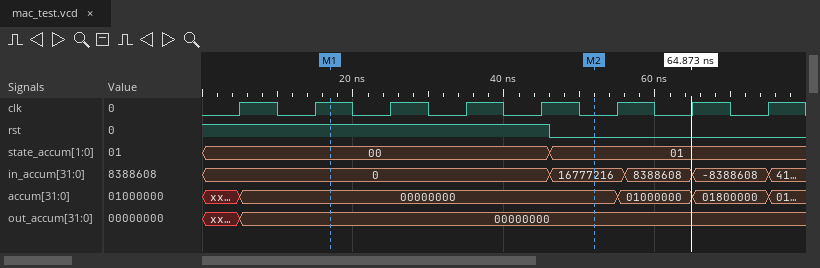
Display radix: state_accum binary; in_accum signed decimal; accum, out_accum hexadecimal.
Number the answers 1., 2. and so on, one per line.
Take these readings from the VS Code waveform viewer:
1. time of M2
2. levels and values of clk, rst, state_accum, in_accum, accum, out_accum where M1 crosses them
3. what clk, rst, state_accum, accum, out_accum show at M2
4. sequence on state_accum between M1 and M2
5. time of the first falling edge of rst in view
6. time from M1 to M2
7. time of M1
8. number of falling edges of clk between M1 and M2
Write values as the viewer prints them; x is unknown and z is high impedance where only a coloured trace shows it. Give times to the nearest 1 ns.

1. 52 ns
2. clk=1, rst=1, state_accum=00, in_accum=0, accum=00000000, out_accum=00000000
3. clk=0, rst=0, state_accum=01, accum=00000000, out_accum=00000000
4. 00, 01
5. 46 ns
6. 35 ns
7. 17 ns
8. 4
